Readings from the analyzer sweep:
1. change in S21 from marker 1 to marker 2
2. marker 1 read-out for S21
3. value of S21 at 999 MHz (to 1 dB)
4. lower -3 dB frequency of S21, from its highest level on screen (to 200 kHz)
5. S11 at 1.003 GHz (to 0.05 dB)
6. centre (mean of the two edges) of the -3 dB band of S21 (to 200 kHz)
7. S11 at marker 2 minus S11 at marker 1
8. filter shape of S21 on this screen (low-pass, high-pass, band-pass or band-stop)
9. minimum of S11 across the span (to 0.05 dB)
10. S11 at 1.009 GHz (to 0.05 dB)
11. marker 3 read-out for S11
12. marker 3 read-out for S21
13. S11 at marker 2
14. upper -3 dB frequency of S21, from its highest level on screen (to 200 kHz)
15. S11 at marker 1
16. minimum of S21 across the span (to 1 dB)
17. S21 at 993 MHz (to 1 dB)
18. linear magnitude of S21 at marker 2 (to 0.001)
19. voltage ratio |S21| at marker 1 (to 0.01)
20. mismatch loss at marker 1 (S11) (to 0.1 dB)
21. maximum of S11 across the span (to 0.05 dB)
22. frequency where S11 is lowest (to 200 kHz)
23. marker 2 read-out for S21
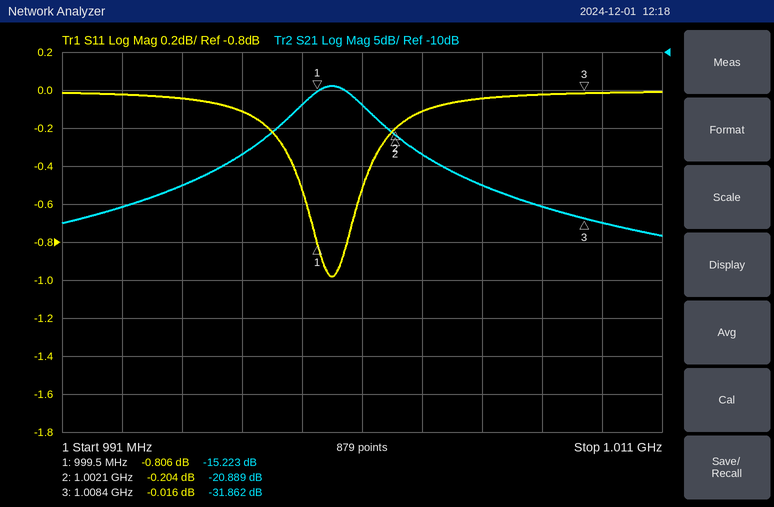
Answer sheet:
-5.666 dB
-15.223 dB
-17 dB
998.8 MHz
-0.10 dB
1.0000 GHz
0.602 dB
band-pass
-1.00 dB
0.00 dB
-0.016 dB
-31.862 dB
-0.204 dB
1.0012 GHz
-0.806 dB
-34 dB
-30 dB
0.090
0.17
7.7 dB
0.00 dB
1.0000 GHz
-20.889 dB
